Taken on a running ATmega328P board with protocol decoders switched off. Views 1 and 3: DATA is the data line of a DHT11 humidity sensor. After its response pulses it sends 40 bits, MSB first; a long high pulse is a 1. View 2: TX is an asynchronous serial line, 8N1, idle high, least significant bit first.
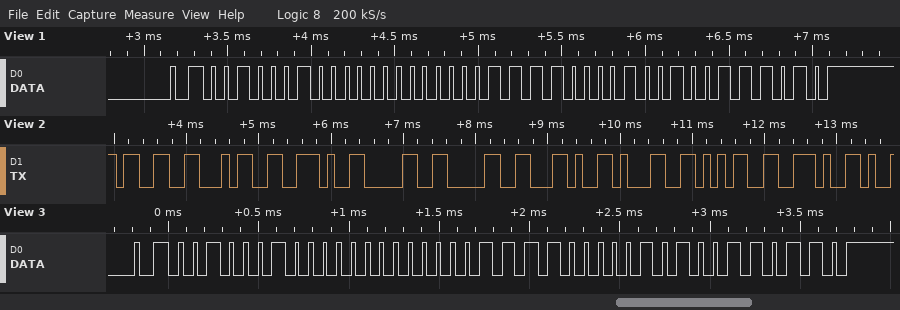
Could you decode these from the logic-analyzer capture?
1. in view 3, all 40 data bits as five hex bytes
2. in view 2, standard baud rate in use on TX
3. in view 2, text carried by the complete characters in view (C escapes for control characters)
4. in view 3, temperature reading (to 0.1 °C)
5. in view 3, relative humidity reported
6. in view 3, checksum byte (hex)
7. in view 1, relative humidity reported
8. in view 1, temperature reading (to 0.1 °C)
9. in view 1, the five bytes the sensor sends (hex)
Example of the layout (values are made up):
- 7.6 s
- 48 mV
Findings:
- 22 00 0F 05 36
- 9600 baud
- "34.00,15."
- 15.5 °C
- 34 %
- 0x36
- 34 %
- 15.9 °C
- 22 00 0F 09 3A
